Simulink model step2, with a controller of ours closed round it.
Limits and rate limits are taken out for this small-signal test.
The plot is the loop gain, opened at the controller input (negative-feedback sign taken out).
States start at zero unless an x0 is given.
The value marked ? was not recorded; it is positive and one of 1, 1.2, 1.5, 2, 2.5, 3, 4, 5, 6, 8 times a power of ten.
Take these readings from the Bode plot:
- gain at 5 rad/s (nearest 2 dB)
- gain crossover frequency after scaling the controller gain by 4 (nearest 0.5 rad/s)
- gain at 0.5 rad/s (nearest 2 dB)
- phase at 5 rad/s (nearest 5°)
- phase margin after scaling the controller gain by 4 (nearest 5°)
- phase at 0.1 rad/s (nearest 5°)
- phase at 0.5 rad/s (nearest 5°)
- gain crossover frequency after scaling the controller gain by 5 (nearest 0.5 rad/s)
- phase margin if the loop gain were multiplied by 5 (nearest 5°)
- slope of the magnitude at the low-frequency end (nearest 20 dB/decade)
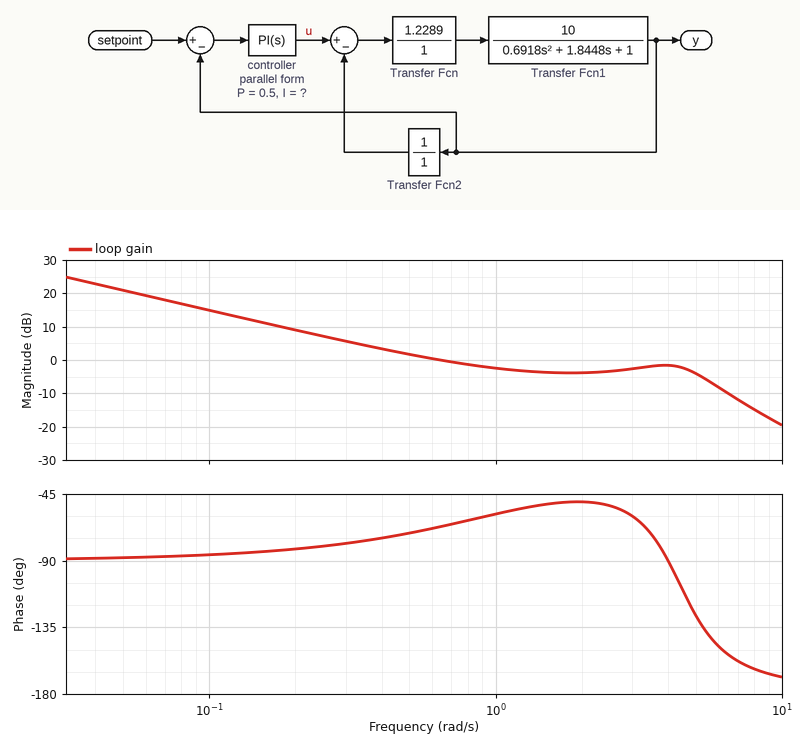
-4 dB
7.0 rad/s
2 dB
-125°
20°
-85°
-70°
7.5 rad/s
20°
-20 dB/decade
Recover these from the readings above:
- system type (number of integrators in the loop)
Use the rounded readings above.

1
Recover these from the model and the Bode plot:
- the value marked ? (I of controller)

0.6
